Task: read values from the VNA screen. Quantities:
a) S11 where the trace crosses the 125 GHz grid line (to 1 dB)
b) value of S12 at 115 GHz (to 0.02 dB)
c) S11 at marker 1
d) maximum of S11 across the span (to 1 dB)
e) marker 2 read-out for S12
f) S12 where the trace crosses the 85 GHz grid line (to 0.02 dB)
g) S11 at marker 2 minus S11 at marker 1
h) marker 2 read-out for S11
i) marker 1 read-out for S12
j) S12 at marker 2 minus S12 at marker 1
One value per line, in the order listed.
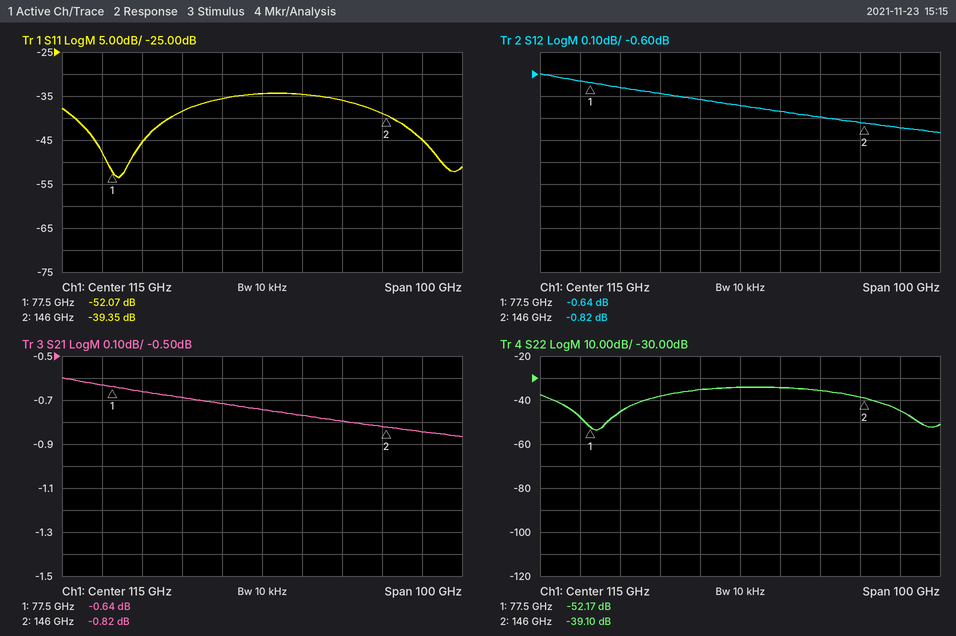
-35 dB
-0.74 dB
-52.07 dB
-34 dB
-0.82 dB
-0.66 dB
12.72 dB
-39.35 dB
-0.64 dB
-0.18 dB
